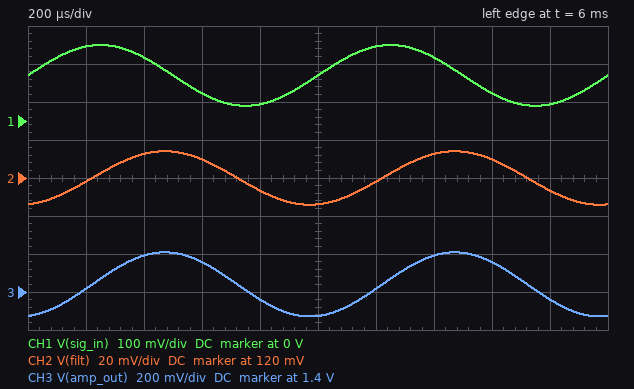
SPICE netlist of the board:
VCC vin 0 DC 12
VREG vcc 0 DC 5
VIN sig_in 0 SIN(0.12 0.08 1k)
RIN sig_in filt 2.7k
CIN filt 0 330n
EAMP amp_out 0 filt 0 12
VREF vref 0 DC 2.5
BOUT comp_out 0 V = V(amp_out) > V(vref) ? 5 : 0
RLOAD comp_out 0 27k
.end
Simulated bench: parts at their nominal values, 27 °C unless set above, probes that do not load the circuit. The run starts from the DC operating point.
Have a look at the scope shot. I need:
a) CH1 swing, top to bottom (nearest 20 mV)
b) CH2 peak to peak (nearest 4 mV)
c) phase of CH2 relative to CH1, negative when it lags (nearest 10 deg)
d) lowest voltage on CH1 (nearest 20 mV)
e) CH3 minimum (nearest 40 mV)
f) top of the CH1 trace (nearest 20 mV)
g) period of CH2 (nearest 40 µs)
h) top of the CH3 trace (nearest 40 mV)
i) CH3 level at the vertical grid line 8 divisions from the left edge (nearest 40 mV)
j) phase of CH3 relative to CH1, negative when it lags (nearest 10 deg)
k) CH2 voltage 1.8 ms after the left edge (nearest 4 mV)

160 mV
28 mV
-80 deg
40 mV
1.28 V
200 mV
1.00 ms
1.60 V
1.56 V
-80 deg
112 mV
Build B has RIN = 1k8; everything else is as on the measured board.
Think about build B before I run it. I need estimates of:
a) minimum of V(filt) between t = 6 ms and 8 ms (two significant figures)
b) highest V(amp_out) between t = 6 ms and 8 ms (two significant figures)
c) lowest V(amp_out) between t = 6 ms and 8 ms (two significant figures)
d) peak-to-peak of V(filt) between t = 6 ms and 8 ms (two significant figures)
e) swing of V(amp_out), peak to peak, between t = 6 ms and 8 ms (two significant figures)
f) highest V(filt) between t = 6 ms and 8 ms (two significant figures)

99 mV
1.7 V
1.2 V
41 mV
500 mV
140 mV
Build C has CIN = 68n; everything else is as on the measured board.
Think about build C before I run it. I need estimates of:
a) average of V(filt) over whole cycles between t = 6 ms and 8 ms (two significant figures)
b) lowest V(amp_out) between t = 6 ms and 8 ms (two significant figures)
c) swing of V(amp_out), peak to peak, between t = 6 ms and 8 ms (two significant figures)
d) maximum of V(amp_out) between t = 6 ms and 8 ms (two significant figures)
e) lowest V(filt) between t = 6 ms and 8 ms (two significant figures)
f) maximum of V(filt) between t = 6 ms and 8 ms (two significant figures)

120 mV
810 mV
1.3 V
2.1 V
68 mV
170 mV
